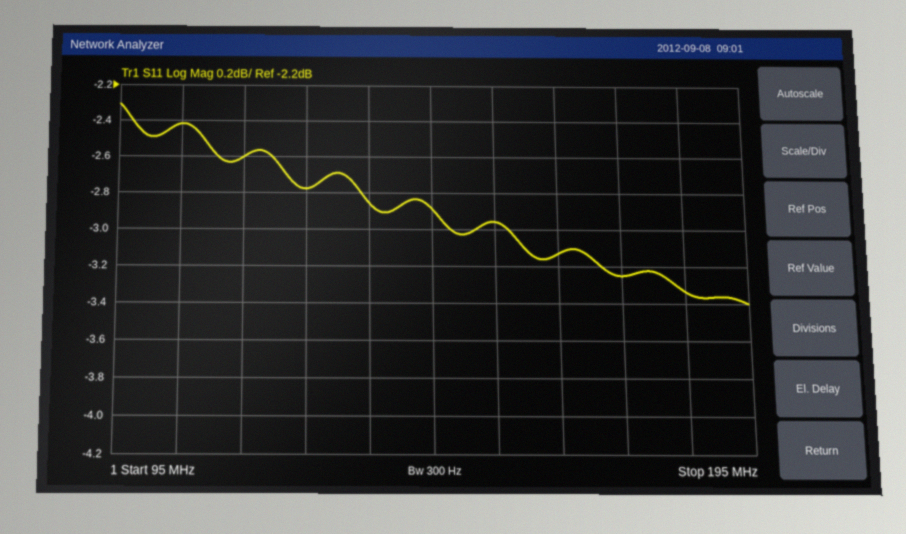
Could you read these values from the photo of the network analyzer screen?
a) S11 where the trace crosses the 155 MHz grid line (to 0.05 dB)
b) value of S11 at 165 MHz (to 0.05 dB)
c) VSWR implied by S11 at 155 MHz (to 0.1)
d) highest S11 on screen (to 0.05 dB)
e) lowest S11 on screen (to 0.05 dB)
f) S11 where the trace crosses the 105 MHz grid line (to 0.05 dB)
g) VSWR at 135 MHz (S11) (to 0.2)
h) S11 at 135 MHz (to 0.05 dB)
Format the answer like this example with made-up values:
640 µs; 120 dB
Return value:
-2.95 dB; -3.15 dB; 5.9; -2.30 dB; -3.40 dB; -2.40 dB; 6.2; -2.85 dB
